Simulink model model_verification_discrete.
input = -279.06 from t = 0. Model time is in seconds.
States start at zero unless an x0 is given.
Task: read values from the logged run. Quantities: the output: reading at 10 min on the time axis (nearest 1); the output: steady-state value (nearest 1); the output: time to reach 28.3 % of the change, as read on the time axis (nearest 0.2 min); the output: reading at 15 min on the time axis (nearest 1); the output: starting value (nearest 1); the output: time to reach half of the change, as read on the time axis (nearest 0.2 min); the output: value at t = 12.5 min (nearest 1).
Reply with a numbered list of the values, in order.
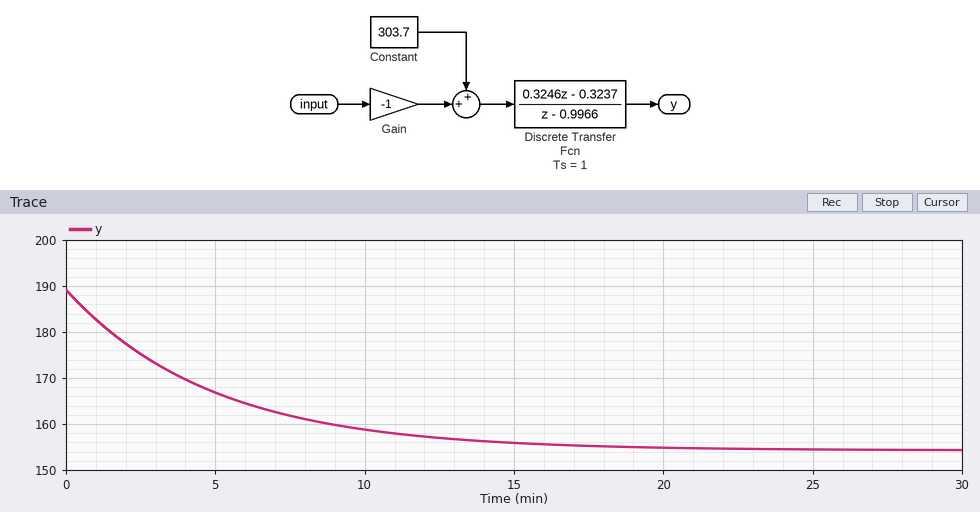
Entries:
1. 159
2. 154
3. 1.6 min
4. 156
5. 189
6. 3.4 min
7. 157
